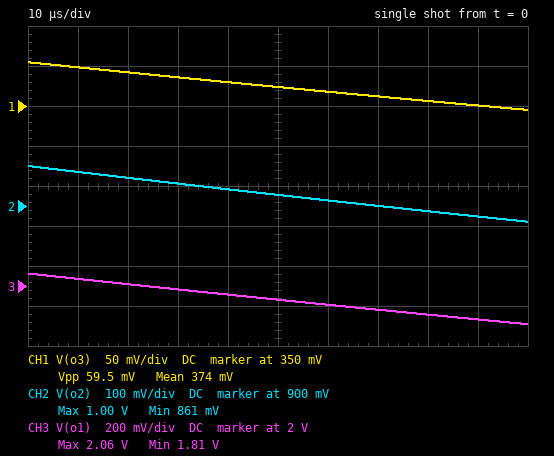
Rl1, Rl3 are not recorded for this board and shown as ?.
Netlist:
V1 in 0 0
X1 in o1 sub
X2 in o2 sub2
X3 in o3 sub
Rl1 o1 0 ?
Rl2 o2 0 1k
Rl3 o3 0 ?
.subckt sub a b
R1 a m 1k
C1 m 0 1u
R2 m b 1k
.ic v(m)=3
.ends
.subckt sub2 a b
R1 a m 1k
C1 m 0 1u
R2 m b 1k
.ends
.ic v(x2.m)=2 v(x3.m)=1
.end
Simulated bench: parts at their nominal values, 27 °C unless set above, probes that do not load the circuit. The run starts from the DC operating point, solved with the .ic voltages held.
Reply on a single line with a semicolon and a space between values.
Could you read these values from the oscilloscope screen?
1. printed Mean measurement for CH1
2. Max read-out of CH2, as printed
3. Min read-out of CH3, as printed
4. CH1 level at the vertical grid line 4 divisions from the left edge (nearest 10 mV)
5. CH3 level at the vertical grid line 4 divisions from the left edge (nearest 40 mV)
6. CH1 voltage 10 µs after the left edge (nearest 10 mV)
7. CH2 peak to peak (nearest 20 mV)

374 mV; 1.00 V; 1.81 V; 380 mV; 1.96 V; 400 mV; 140 mV
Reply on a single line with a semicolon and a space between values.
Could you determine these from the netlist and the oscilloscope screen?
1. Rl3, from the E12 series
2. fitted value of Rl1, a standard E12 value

680 Ω; 2.2 kΩ
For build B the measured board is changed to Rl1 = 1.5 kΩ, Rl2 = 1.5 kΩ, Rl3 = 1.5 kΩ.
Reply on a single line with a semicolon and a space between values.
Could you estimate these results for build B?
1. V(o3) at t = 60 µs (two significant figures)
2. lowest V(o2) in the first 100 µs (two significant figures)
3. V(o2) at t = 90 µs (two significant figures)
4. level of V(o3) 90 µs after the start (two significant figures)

550 mV; 1.0 V; 1.1 V; 530 mV
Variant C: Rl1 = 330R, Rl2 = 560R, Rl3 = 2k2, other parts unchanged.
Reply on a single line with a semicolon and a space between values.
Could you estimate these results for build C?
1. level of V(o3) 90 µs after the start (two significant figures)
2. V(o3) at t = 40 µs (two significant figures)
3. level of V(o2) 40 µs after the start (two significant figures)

610 mV; 650 mV; 670 mV
